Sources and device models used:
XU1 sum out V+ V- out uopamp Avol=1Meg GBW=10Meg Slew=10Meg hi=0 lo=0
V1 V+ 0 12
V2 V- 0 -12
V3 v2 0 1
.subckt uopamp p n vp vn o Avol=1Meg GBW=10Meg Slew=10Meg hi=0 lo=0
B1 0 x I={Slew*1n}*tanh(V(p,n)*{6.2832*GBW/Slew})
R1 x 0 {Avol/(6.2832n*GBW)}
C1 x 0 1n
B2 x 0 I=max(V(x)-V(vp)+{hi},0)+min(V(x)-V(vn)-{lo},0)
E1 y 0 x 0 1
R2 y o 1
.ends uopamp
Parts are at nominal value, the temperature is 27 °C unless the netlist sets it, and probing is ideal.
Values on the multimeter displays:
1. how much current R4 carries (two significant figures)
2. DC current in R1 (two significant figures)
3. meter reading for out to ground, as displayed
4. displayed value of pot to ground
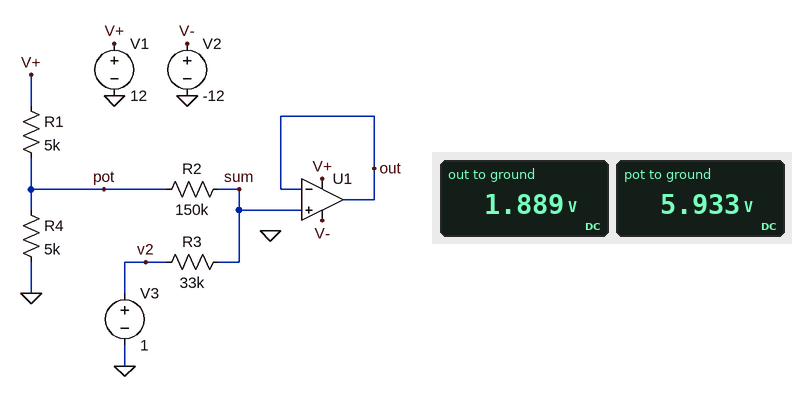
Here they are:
1.2 mA
1.2 mA
1.889 V
5.933 V
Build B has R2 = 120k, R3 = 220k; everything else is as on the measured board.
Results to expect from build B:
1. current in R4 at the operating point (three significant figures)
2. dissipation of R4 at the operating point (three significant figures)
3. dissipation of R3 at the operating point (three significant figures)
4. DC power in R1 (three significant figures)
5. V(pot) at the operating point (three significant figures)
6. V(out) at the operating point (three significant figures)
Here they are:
1.19 mA
7.11 mW
46.9 µW
7.29 mW
5.96 V
4.21 V
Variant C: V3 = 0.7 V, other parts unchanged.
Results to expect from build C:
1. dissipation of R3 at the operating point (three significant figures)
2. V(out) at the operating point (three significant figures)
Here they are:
26.9 µW
1.64 V
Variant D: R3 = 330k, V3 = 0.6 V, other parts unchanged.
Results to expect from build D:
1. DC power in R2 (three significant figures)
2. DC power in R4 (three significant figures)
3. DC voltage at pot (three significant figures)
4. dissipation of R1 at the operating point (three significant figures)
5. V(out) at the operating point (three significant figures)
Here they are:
18.8 µW
7.13 mW
5.97 V
7.27 mW
4.29 V
